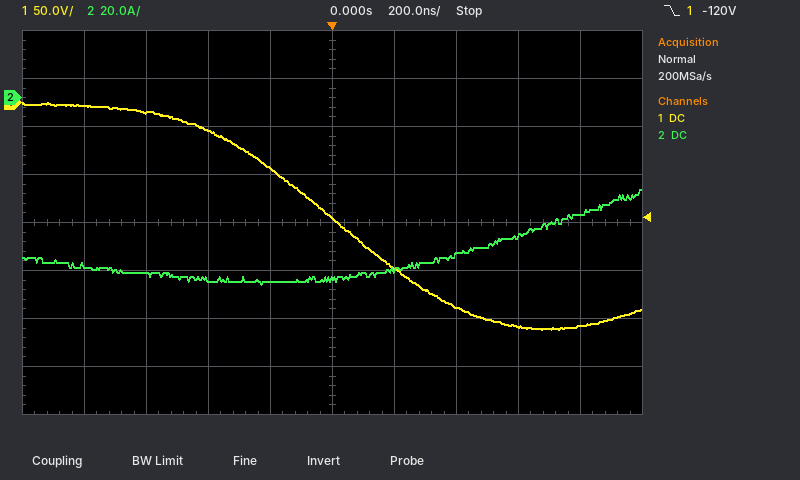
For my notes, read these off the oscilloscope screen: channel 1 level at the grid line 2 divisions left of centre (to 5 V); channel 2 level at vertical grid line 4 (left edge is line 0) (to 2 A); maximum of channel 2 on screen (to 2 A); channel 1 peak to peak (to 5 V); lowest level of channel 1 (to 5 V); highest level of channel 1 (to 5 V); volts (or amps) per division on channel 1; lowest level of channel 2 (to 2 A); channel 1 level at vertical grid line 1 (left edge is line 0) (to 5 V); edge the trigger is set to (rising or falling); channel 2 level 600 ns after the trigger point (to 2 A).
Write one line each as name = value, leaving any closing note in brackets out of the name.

channel 1 level at the grid line 2 divisions left of centre = -30 V
channel 2 level at vertical grid line 4 (left edge is line 0) = -76 A
maximum of channel 2 on screen = -38 A
channel 1 peak to peak = 235 V
lowest level of channel 1 = -235 V
highest level of channel 1 = 0 V
volts (or amps) per division on channel 1 = 50 V
lowest level of channel 2 = -78 A
channel 1 level at vertical grid line 1 (left edge is line 0) = -5 V
edge the trigger is set to = falling
channel 2 level 600 ns after the trigger point = -58 A
